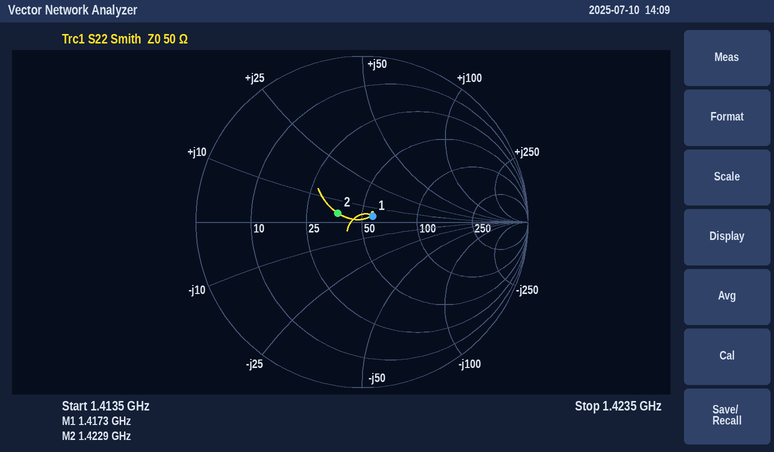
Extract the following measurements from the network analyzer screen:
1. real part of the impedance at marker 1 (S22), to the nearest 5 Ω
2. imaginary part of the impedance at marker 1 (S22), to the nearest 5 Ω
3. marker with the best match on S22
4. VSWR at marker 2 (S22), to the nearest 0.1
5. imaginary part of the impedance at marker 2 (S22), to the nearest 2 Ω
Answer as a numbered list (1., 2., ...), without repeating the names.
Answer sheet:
1. 55 Ω
2. +5 Ω
3. marker 1
4. 1.4
5. +4 Ω
